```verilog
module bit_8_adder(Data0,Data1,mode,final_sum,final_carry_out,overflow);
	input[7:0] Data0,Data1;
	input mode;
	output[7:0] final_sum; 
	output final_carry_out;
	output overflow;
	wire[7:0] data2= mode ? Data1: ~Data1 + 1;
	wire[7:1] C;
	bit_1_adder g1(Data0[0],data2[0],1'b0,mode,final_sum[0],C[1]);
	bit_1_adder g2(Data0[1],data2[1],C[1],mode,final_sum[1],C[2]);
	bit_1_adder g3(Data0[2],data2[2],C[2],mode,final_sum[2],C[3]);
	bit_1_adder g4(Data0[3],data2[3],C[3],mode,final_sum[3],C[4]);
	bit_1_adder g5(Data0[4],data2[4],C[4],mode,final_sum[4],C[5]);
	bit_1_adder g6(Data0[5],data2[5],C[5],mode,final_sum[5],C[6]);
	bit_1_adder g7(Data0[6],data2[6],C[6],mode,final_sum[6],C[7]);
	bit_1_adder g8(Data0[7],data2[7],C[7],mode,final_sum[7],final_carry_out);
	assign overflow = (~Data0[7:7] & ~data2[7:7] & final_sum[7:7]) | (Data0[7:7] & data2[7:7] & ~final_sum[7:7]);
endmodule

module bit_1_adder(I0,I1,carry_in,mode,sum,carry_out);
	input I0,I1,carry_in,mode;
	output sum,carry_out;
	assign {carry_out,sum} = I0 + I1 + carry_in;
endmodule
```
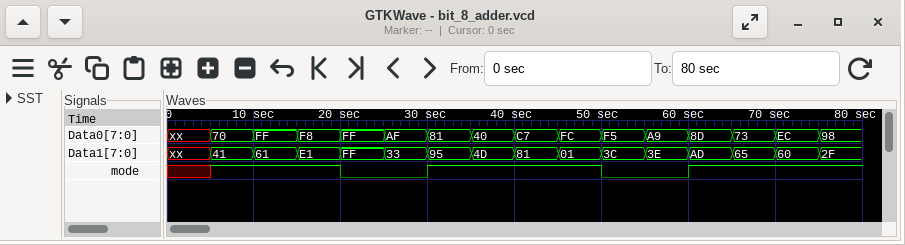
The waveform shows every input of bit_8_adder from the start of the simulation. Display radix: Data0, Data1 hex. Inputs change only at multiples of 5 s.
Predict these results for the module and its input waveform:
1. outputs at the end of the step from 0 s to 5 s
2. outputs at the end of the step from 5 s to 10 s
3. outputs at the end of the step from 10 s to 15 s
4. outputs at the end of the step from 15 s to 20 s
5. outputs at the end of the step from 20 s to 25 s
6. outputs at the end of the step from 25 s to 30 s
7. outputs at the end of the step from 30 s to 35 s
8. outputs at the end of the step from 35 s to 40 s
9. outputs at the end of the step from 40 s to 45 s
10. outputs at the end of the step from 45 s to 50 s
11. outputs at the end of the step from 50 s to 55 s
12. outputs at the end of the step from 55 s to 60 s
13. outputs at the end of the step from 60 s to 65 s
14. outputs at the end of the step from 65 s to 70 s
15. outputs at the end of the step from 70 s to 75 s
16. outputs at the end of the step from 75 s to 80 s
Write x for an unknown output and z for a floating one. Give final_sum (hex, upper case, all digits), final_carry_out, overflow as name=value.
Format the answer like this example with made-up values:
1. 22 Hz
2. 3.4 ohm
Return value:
1. final_sum=x, final_carry_out=x, overflow=x
2. final_sum=B1, final_carry_out=0, overflow=1
3. final_sum=60, final_carry_out=1, overflow=0
4. final_sum=D9, final_carry_out=1, overflow=0
5. final_sum=00, final_carry_out=1, overflow=0
6. final_sum=7C, final_carry_out=1, overflow=1
7. final_sum=16, final_carry_out=1, overflow=1
8. final_sum=8D, final_carry_out=0, overflow=1
9. final_sum=48, final_carry_out=1, overflow=1
10. final_sum=FD, final_carry_out=0, overflow=0
11. final_sum=B9, final_carry_out=1, overflow=0
12. final_sum=6B, final_carry_out=1, overflow=1
13. final_sum=3A, final_carry_out=1, overflow=1
14. final_sum=D8, final_carry_out=0, overflow=1
15. final_sum=4C, final_carry_out=1, overflow=0
16. final_sum=C7, final_carry_out=0, overflow=0
